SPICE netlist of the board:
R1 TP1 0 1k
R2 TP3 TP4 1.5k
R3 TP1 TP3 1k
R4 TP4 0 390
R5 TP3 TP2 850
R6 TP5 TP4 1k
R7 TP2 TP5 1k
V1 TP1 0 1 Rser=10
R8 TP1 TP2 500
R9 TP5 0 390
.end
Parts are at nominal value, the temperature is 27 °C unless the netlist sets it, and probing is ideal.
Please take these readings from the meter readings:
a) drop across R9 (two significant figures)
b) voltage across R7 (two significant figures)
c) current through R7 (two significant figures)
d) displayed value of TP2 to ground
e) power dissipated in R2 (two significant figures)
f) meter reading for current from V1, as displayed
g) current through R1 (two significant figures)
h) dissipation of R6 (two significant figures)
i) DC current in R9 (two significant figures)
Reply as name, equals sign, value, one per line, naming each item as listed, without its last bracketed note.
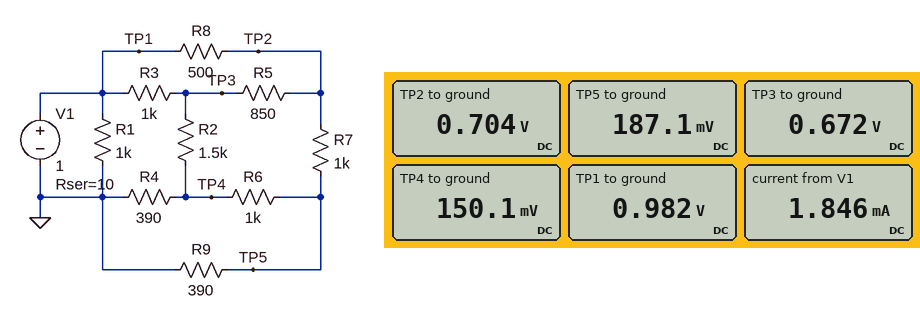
drop across R9 = 190 mV
voltage across R7 = 520 mV
current through R7 = 520 µA
displayed value of TP2 to ground = 0.704 V
power dissipated in R2 = 180 µW
meter reading for current from V1, as displayed = 1.846 mA
current through R1 = 980 µA
dissipation of R6 = 1.4 µW
DC current in R9 = 480 µA
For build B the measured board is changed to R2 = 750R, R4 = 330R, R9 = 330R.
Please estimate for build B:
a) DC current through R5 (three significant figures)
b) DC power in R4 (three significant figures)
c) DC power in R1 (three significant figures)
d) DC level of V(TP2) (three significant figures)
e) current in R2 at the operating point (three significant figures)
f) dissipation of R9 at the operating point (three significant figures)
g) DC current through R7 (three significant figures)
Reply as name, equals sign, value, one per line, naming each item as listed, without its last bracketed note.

DC current through R5 = 118 µA
DC power in R4 = 90.4 µW
DC power in R1 = 960 µW
DC level of V(TP2) = 670 mV
current in R2 at the operating point = 529 µA
dissipation of R9 at the operating point = 85.0 µW
DC current through R7 = 502 µA
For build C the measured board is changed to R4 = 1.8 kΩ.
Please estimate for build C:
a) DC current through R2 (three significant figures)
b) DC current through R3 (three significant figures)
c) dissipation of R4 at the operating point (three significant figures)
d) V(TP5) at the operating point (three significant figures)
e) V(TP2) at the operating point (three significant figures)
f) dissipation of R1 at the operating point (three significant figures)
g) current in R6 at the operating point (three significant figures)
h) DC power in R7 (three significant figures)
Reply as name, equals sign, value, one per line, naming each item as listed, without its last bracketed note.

DC current through R2 = 268 µA
DC current through R3 = 260 µA
dissipation of R4 at the operating point = 56.9 µW
V(TP5) at the operating point = 230 mV
V(TP2) at the operating point = 729 mV
dissipation of R1 at the operating point = 965 µW
current in R6 at the operating point = 90.3 µA
DC power in R7 = 249 µW
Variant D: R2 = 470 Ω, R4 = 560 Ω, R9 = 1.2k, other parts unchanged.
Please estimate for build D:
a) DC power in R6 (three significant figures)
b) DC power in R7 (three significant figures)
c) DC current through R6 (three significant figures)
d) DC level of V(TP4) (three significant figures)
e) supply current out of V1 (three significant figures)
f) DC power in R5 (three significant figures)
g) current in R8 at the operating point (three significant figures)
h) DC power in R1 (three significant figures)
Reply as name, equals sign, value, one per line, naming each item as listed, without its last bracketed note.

DC power in R6 = 1.73 µW
DC power in R7 = 124 µW
DC current through R6 = 41.6 µA
DC level of V(TP4) = 331 mV
supply current out of V1 = 1.88 mA
DC power in R5 = 21.5 µW
current in R8 at the operating point = 512 µA
DC power in R1 = 963 µW
